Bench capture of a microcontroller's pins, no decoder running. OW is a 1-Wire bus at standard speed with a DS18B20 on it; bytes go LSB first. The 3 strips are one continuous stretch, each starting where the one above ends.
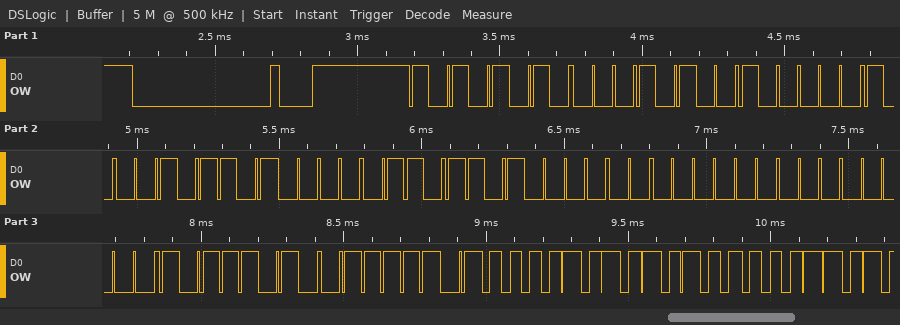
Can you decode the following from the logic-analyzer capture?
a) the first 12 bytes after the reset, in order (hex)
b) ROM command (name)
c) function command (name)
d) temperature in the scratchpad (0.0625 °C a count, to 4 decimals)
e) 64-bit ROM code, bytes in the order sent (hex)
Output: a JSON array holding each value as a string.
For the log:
["55 28 41 B4 60 0B 00 00 5D BE 50 05", "Match ROM", "Read Scratchpad", "85.0000 °C", "28 41 B4 60 0B 00 00 5D"]
